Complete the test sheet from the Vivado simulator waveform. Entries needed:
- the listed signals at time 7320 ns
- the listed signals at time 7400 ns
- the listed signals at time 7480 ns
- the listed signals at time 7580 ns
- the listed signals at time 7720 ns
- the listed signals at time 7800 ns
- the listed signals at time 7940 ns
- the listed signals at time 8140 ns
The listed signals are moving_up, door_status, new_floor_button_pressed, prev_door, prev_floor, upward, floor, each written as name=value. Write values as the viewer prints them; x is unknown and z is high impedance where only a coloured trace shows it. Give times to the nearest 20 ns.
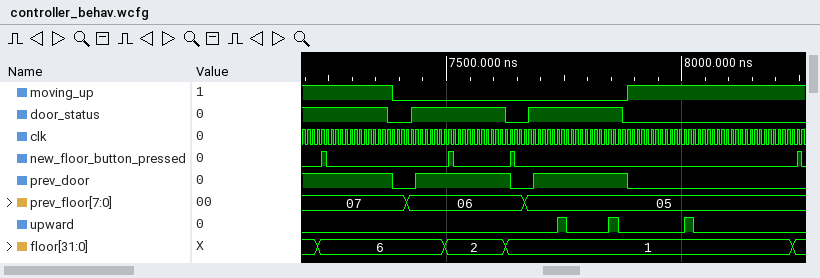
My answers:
moving_up=1, door_status=1, new_floor_button_pressed=0, prev_door=1, prev_floor=07, upward=0, floor=6
moving_up=0, door_status=0, new_floor_button_pressed=0, prev_door=0, prev_floor=07, upward=0, floor=6
moving_up=0, door_status=1, new_floor_button_pressed=0, prev_door=1, prev_floor=06, upward=0, floor=6
moving_up=0, door_status=1, new_floor_button_pressed=0, prev_door=1, prev_floor=06, upward=0, floor=2
moving_up=0, door_status=1, new_floor_button_pressed=0, prev_door=1, prev_floor=05, upward=0, floor=1
moving_up=0, door_status=1, new_floor_button_pressed=0, prev_door=1, prev_floor=05, upward=0, floor=1
moving_up=1, door_status=0, new_floor_button_pressed=0, prev_door=0, prev_floor=05, upward=0, floor=1
moving_up=1, door_status=0, new_floor_button_pressed=0, prev_door=0, prev_floor=05, upward=0, floor=1
